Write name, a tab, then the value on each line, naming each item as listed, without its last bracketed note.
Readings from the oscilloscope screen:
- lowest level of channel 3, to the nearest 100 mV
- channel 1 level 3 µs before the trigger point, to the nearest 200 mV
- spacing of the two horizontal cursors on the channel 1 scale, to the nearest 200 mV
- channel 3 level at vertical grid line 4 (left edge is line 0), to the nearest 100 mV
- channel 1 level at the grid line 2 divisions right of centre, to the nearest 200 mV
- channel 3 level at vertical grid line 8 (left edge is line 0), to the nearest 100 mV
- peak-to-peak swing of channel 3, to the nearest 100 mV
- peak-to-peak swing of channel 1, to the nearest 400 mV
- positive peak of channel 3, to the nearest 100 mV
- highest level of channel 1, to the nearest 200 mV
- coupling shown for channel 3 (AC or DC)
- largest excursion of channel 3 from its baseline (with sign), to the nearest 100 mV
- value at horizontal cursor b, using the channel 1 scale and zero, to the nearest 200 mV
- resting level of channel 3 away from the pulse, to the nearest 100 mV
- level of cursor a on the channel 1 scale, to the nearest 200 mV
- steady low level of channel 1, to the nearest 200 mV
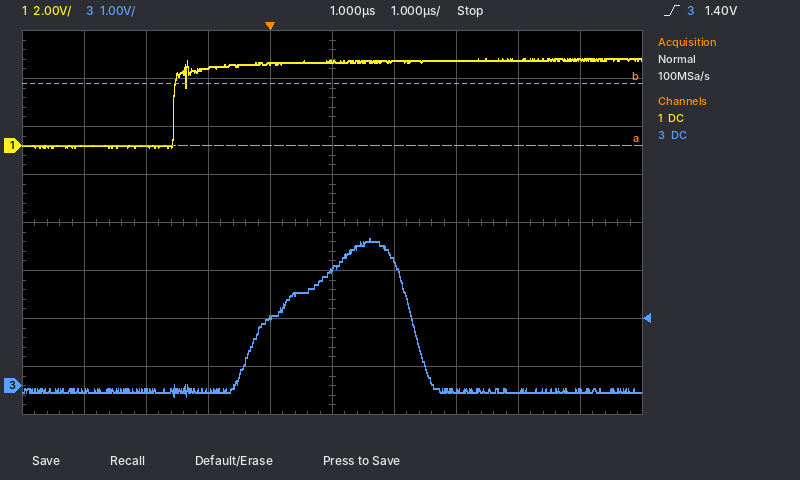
lowest level of channel 3, to the nearest 100 mV	-200 mV
channel 1 level 3 µs before the trigger point, to the nearest 200 mV	0.0 V
spacing of the two horizontal cursors on the channel 1 scale, to the nearest 200 mV	2.6 V
channel 3 level at vertical grid line 4 (left edge is line 0), to the nearest 100 mV	1.4 V
channel 1 level at the grid line 2 divisions right of centre, to the nearest 200 mV	3.6 V
channel 3 level at vertical grid line 8 (left edge is line 0), to the nearest 100 mV	-100 mV
peak-to-peak swing of channel 3, to the nearest 100 mV	3.3 V
peak-to-peak swing of channel 1, to the nearest 400 mV	3.6 V
positive peak of channel 3, to the nearest 100 mV	3.1 V
highest level of channel 1, to the nearest 200 mV	3.6 V
coupling shown for channel 3	DC
largest excursion of channel 3 from its baseline (with sign), to the nearest 100 mV	+3.2 V
value at horizontal cursor b, using the channel 1 scale and zero, to the nearest 200 mV	2.6 V
resting level of channel 3 away from the pulse, to the nearest 100 mV	-100 mV
level of cursor a on the channel 1 scale, to the nearest 200 mV	0.0 V
steady low level of channel 1, to the nearest 200 mV	0.0 V
